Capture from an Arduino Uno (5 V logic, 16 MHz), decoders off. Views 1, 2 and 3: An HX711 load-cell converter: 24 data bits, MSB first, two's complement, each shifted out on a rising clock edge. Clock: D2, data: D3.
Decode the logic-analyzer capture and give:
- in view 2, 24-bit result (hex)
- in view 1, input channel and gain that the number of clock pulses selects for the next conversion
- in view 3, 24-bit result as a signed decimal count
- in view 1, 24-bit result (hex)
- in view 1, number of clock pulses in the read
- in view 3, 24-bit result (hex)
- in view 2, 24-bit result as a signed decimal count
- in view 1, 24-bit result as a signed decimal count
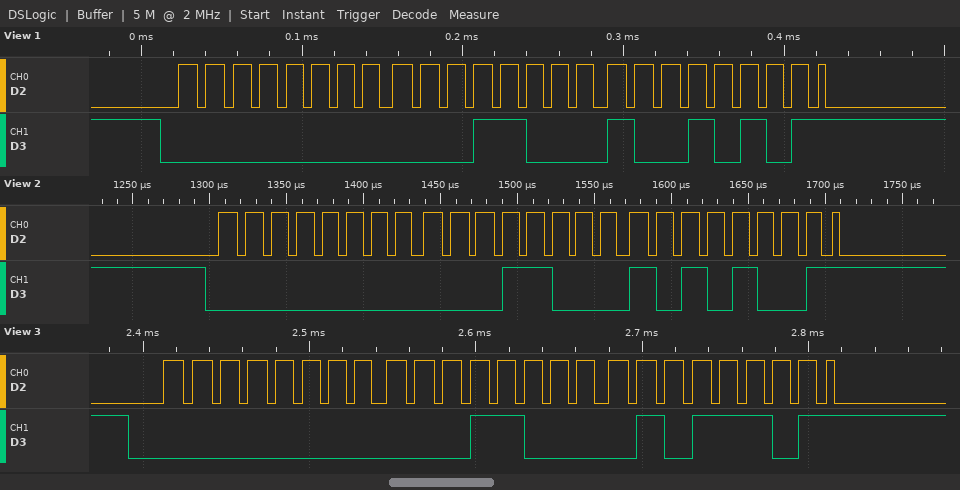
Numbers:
0x0018A9
channel A, gain 128
6237
0x001895
25
0x00185D
6313
6293
